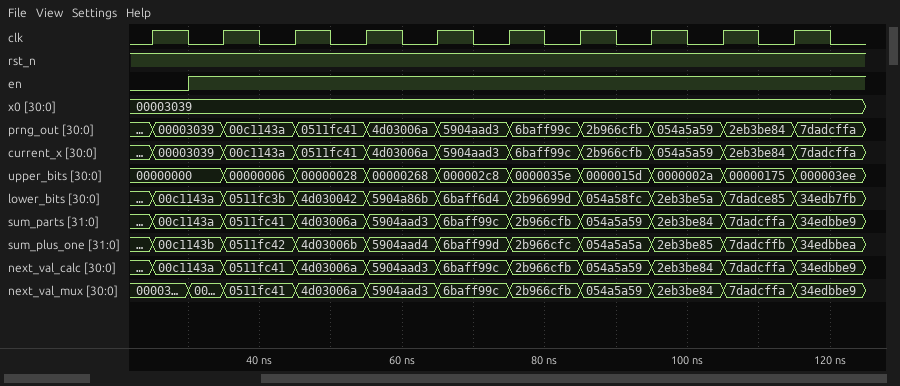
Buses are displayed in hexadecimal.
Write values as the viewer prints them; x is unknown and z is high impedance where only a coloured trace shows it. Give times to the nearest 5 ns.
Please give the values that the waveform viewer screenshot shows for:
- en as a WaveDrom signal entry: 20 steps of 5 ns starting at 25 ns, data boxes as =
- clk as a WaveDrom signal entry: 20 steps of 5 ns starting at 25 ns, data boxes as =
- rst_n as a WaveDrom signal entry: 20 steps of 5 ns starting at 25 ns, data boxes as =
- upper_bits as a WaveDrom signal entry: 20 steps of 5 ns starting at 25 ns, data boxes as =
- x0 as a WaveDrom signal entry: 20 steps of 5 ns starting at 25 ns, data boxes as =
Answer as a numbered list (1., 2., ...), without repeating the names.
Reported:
1. {name: 'en', wave: '01..................'}
2. {name: 'clk', wave: '10101010101010101010'}
3. {name: 'rst_n', wave: '1...................'}
4. {name: 'upper_bits', wave: '=.=.=.=.=.=.=.=.=.=.', data: '00000000 00000006 00000028 00000268 000002c8 0000035e 0000015d 0000002a 00000175 000003ee'}
5. {name: 'x0', wave: '=...................', data: '00003039'}
